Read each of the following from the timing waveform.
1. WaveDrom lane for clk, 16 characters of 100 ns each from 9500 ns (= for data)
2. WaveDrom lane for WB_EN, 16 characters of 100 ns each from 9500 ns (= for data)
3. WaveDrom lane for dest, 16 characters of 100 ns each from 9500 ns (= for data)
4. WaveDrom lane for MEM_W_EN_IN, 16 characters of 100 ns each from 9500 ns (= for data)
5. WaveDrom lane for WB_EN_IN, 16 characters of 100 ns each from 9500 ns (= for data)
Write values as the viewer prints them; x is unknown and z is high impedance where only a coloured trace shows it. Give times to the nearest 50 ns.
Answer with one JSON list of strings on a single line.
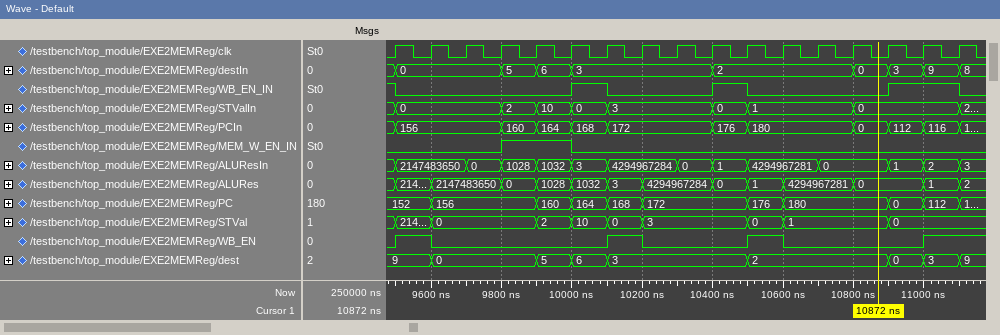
["{name: 'clk', wave: 'p...............'}", "{name: 'WB_EN', wave: '10....10..10...1'}", "{name: 'dest', wave: '==..===...=...==', data: '9 0 5 6 3 2 0 3'}", "{name: 'MEM_W_EN_IN', wave: '0..1.0..........'}", "{name: 'WB_EN_IN', wave: '0....10..10...1.'}"]
